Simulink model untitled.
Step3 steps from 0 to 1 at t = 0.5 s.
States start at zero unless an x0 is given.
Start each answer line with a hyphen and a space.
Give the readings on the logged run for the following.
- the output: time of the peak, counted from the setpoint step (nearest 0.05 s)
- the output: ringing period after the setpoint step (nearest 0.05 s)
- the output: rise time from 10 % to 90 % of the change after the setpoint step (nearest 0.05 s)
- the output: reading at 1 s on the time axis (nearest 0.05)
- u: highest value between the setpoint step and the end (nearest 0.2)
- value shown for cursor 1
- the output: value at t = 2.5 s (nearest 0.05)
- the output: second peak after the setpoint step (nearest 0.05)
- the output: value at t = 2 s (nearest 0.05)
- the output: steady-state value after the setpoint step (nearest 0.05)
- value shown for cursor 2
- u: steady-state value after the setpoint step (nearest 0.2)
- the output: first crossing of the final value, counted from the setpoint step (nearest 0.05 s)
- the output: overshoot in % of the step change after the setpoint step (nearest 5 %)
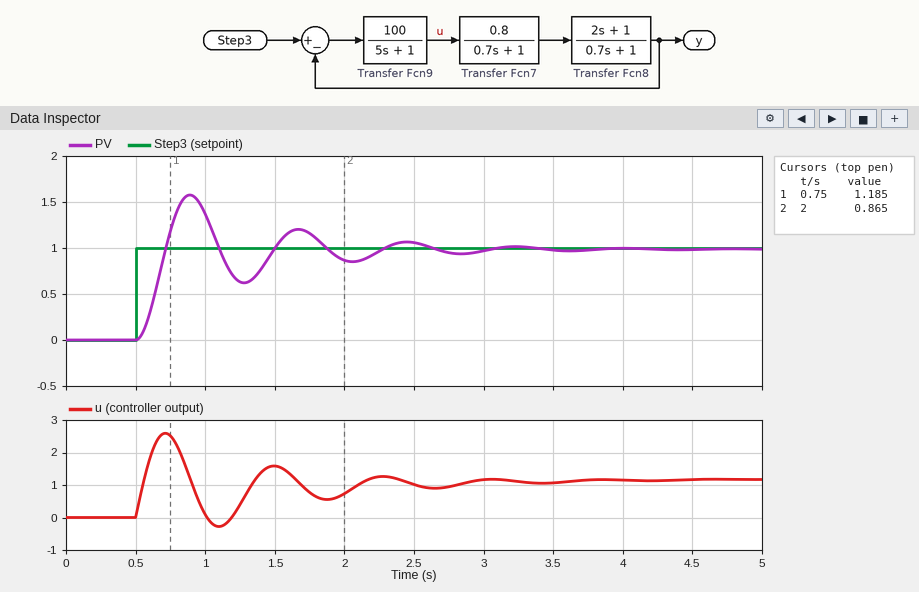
- 0.40 s
- 0.80 s
- 0.15 s
- 1.35
- 2.6
- 1.185
- 1.05
- 1.20
- 0.85
- 1.00
- 0.865
- 1.2
- 0.20 s
- 60 %
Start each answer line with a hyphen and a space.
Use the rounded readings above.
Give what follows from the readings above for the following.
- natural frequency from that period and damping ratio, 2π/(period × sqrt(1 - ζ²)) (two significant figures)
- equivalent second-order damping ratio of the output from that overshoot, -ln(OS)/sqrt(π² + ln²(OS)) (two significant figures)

- 8.0 rad/s
- 0.16
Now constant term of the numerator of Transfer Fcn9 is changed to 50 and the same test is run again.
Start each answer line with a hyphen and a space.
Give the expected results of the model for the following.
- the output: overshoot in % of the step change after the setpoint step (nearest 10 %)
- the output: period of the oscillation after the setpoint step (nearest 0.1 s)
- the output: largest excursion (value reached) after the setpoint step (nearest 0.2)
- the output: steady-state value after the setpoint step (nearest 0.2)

- 50 %
- 1.1 s
- 1.4
- 1.0
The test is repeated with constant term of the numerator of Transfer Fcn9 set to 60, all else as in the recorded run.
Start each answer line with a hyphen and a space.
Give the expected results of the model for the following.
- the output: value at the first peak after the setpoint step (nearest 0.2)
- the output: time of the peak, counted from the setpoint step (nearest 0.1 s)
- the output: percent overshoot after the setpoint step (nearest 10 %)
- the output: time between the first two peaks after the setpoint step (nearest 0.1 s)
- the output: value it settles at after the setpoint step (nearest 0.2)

- 1.4
- 0.5 s
- 50 %
- 1.0 s
- 1.0
